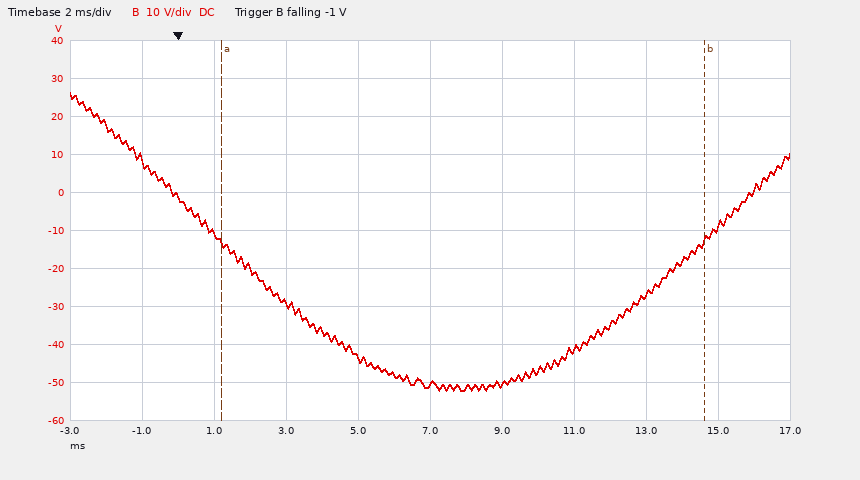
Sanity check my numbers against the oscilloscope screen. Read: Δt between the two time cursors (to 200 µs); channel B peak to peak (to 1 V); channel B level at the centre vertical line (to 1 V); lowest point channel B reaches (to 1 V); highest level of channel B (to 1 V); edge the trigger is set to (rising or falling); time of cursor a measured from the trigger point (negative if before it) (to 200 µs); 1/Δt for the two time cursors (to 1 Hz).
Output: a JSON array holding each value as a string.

["13.4 ms", "78 V", "-50 V", "-52 V", "26 V", "falling", "+1.2 ms", "75 Hz"]
